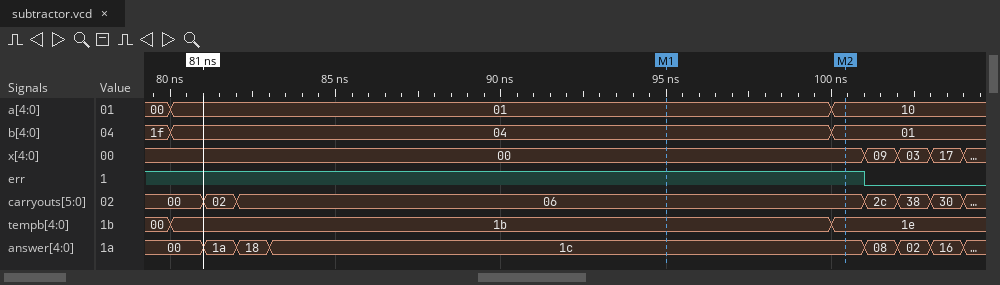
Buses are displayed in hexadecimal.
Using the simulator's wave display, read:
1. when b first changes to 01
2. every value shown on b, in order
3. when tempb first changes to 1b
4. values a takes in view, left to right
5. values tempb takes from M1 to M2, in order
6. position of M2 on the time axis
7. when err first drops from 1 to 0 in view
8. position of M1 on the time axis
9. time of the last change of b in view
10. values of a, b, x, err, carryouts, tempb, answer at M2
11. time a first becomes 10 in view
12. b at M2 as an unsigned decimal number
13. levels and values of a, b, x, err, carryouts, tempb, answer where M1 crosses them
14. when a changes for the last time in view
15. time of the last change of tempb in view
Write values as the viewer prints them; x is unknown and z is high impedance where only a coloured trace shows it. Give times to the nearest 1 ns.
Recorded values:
100 ns
1f, 04, 01
80 ns
00, 01, 10
1b, 1e
100 ns
101 ns
95 ns
100 ns
a=10, b=01, x=00, err=1, carryouts=06, tempb=1e, answer=1c
100 ns
1
a=01, b=04, x=00, err=1, carryouts=06, tempb=1b, answer=1c
100 ns
100 ns
